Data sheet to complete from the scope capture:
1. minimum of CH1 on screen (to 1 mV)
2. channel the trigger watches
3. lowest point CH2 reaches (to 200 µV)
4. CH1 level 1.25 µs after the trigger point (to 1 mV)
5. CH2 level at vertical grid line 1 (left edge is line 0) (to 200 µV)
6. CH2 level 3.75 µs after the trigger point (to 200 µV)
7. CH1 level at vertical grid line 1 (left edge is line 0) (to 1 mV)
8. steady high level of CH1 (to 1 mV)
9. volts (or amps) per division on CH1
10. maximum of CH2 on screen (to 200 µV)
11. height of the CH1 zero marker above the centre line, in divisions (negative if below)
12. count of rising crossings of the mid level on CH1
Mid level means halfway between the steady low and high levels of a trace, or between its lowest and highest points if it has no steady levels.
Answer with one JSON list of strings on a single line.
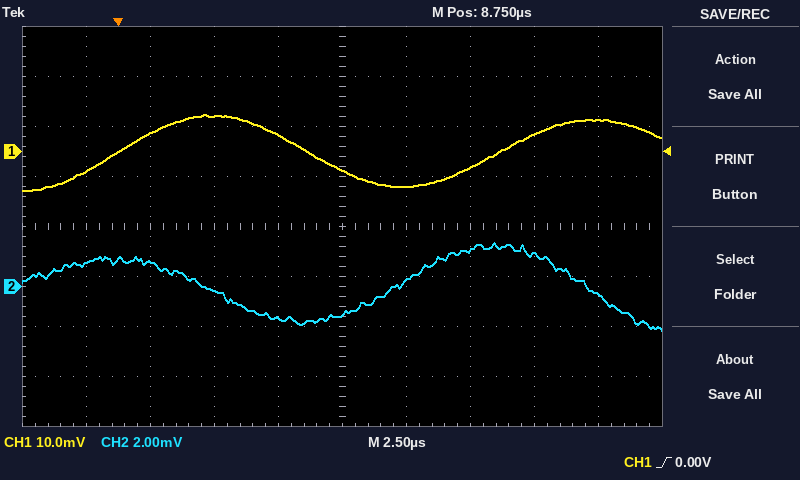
["-8 mV", "CH1", "-1.8 mV", "4 mV", "1.0 mV", "-200 µV", "-4 mV", "6 mV", "10 mV", "1.8 mV", "+1.5 div", "2"]
